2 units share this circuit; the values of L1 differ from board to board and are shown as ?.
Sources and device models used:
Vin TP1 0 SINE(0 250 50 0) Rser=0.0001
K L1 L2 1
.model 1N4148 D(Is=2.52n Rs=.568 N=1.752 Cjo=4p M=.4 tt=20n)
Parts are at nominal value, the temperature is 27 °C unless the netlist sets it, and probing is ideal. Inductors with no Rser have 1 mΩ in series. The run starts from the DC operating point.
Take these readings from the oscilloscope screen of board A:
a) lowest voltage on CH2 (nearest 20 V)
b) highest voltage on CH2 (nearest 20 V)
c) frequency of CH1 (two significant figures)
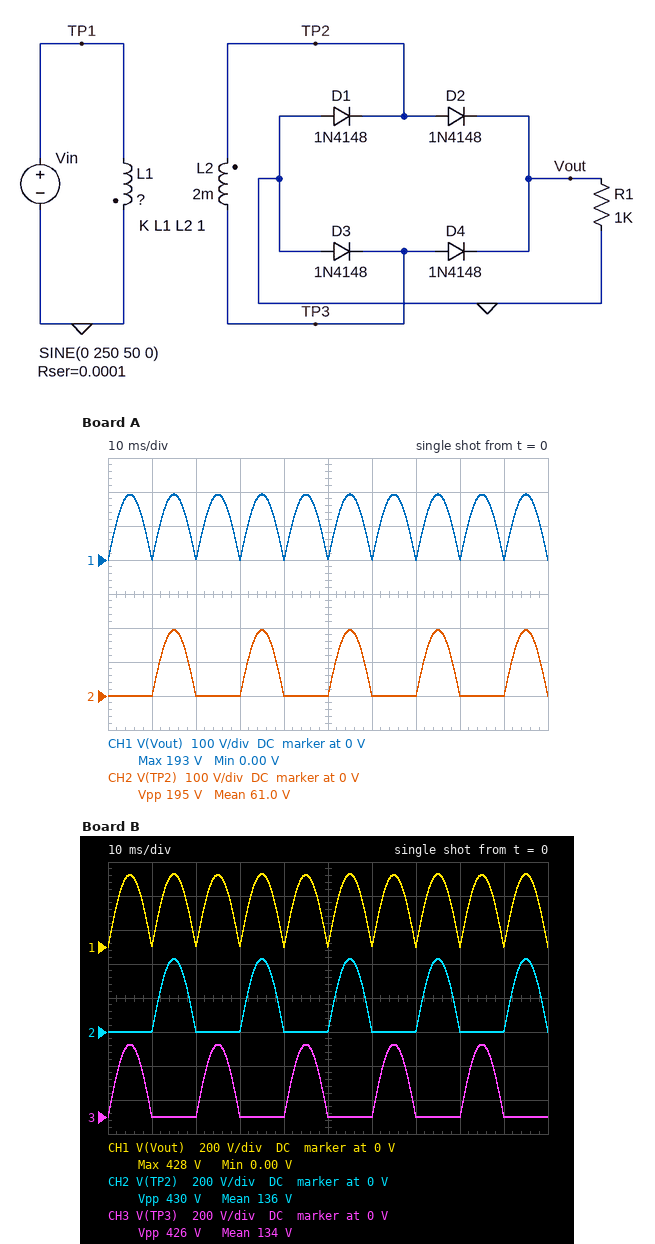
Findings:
0 V
200 V
100 Hz
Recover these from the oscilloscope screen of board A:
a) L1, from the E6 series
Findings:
3.3 mH
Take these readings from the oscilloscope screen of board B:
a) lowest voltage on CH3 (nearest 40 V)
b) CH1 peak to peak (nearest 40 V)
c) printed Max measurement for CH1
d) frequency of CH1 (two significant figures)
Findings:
0 V
440 V
428 V
100 Hz
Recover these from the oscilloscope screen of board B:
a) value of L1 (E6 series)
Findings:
680 µH
